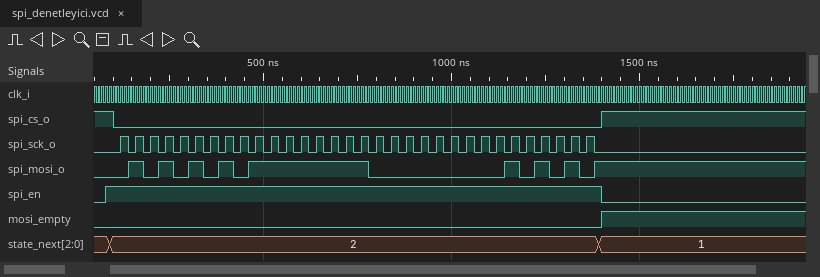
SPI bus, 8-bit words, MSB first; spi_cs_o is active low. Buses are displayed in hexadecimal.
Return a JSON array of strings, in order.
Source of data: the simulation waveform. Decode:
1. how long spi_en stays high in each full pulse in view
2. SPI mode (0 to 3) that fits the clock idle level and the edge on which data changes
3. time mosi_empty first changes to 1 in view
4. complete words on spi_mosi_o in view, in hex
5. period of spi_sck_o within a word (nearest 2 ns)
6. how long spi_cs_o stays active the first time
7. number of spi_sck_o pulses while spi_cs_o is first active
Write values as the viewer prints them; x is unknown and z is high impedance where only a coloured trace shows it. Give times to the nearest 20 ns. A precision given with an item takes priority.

["1320 ns", "0", "1400 ns", "55, 7F, 80, 2A", "40 ns", "1300 ns", "32"]
